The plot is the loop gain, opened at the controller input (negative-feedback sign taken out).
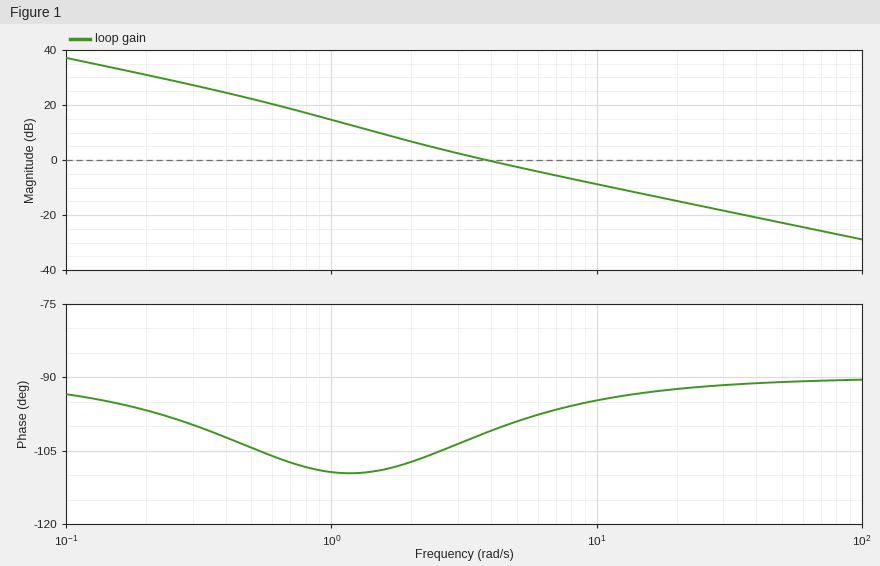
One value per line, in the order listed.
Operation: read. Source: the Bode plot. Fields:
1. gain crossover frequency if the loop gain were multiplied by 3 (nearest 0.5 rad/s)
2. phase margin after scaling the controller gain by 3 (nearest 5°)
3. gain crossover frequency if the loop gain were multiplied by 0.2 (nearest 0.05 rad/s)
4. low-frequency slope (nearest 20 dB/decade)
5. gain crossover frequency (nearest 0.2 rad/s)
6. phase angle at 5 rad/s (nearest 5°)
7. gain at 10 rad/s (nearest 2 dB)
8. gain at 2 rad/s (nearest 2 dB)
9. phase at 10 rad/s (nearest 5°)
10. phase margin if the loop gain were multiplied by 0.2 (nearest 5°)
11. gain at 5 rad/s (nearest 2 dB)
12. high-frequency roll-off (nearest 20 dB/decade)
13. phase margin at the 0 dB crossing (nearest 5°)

11.0 rad/s
85°
1.05 rad/s
-20 dB/decade
3.8 rad/s
-100°
-8 dB
6 dB
-95°
70°
-2 dB
-20 dB/decade
80°
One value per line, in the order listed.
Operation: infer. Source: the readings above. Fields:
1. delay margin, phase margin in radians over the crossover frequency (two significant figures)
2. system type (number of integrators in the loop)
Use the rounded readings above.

0.37 s
1
